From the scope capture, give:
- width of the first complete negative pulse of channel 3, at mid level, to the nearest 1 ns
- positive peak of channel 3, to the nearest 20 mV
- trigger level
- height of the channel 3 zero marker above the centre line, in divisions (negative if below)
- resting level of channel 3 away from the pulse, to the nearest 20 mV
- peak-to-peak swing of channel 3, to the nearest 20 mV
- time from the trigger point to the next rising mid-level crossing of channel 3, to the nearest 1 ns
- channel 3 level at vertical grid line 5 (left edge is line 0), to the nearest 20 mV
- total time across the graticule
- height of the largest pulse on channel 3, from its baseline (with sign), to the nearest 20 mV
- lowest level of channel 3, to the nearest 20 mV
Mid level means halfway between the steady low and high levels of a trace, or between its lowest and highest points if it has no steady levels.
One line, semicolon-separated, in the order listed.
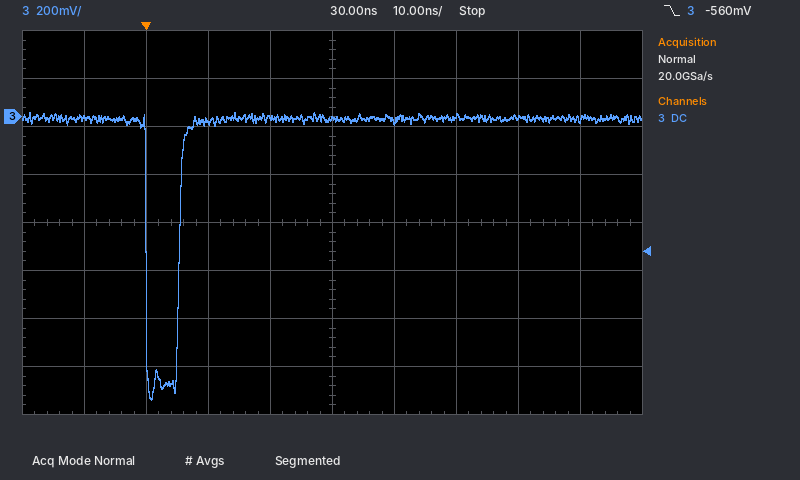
5 ns; 20 mV; -560 mV; +2.2 div; 0 mV; 1.20 V; 5 ns; 0 mV; 100 ns; -1.18 V; -1.18 V
